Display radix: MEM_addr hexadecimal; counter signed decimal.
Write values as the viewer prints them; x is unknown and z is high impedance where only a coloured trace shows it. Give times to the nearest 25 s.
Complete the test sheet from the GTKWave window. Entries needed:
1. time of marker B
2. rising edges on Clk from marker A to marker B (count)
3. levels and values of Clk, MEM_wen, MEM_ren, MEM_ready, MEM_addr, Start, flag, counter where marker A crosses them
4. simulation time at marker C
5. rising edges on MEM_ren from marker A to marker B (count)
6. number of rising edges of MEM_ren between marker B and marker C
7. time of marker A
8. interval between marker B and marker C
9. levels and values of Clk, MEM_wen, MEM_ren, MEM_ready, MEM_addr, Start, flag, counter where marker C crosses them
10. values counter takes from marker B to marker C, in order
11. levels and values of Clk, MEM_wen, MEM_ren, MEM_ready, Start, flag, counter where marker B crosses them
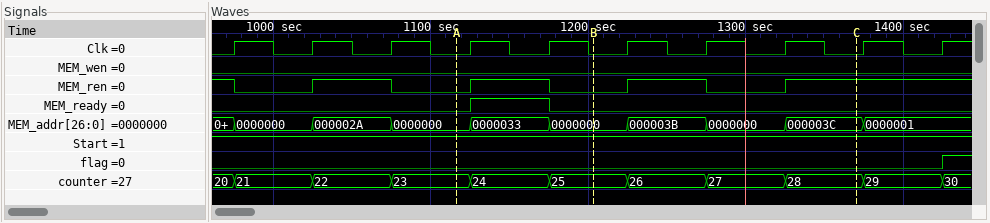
1200 s
2
Clk=0, MEM_wen=0, MEM_ren=0, MEM_ready=0, MEM_addr=0000000, Start=1, flag=0, counter=23
1375 s
1
2
1125 s
175 s
Clk=0, MEM_wen=0, MEM_ren=1, MEM_ready=0, MEM_addr=000003C, Start=1, flag=0, counter=28
25, 26, 27, 28
Clk=0, MEM_wen=0, MEM_ren=0, MEM_ready=0, Start=1, flag=0, counter=25
